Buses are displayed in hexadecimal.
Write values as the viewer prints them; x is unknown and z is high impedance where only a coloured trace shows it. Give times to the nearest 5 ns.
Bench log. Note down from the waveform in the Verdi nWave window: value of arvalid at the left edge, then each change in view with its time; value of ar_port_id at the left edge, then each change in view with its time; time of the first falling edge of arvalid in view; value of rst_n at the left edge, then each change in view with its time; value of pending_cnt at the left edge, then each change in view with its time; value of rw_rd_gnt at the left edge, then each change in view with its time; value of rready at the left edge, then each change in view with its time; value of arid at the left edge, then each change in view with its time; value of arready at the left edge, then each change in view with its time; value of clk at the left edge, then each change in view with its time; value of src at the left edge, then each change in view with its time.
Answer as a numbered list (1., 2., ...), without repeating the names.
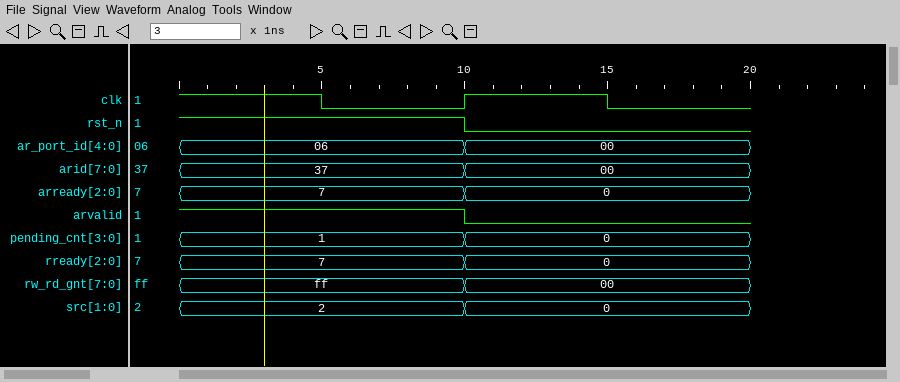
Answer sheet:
1. 1, 0 at 10 ns
2. 06, 00 at 10 ns
3. 10 ns
4. 1, 0 at 10 ns
5. 1, 0 at 10 ns
6. ff, 00 at 10 ns
7. 7, 0 at 10 ns
8. 37, 00 at 10 ns
9. 7, 0 at 10 ns
10. 1, 0 at 5 ns, 1 at 10 ns, 0 at 15 ns
11. 2, 0 at 10 ns
